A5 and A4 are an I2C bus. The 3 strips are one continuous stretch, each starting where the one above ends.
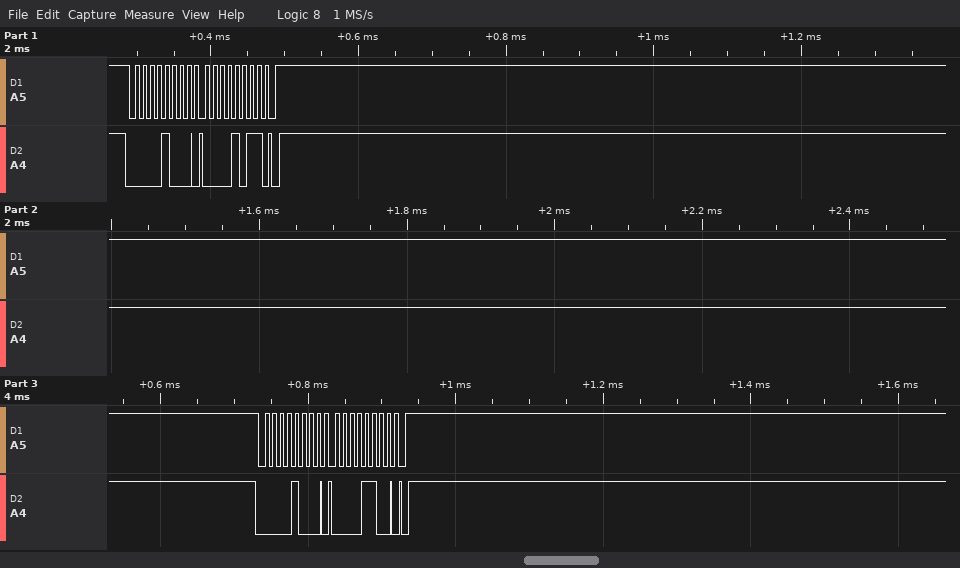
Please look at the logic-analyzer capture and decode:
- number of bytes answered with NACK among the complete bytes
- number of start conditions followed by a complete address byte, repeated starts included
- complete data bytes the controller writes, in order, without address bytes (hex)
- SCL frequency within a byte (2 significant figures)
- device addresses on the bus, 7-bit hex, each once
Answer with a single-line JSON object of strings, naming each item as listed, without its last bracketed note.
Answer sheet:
{"number of bytes answered with NACK among the complete bytes": "0", "number of start conditions followed by a complete address byte, repeated starts included": "2", "complete data bytes the controller writes, in order, without address bytes": "0B 0C", "SCL frequency within a byte": "100 kHz", "device addresses on the bus, 7-bit hex, each once": "0x04"}
